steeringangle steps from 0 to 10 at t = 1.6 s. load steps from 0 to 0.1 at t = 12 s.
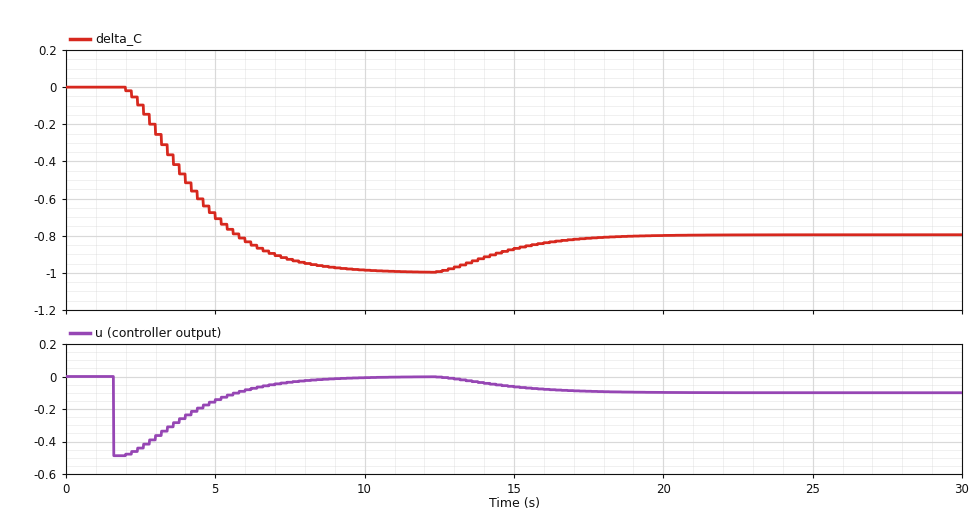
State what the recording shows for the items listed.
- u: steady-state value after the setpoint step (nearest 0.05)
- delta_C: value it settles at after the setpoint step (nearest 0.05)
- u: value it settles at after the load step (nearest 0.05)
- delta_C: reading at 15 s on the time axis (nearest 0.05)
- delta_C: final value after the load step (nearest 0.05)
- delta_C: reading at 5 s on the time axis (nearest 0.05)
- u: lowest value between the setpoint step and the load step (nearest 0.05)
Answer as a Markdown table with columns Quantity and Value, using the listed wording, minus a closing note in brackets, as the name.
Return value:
| Quantity | Value |
|---|---|
| u: steady-state value after the setpoint step | 0.00 |
| delta_C: value it settles at after the setpoint step | -1.00 |
| u: value it settles at after the load step | -0.10 |
| delta_C: reading at 15 s on the time axis | -0.85 |
| delta_C: final value after the load step | -0.80 |
| delta_C: reading at 5 s on the time axis | -0.70 |
| u: lowest value between the setpoint step and the load step | -0.50 |
